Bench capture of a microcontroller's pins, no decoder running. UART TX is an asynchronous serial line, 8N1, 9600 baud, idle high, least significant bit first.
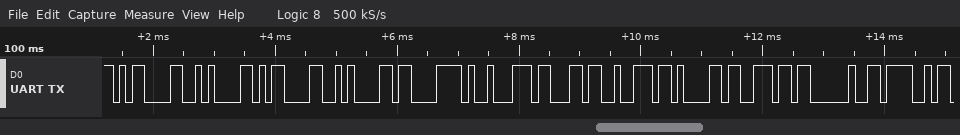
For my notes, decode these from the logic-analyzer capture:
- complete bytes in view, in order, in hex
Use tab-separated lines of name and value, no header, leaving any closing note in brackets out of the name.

complete bytes in view, in order, in hex	0x0D 0x0A 0x0D 0x0A 0xC3 0x89 0x63 0x72 0x61 0x6E 0x20 0x4F
